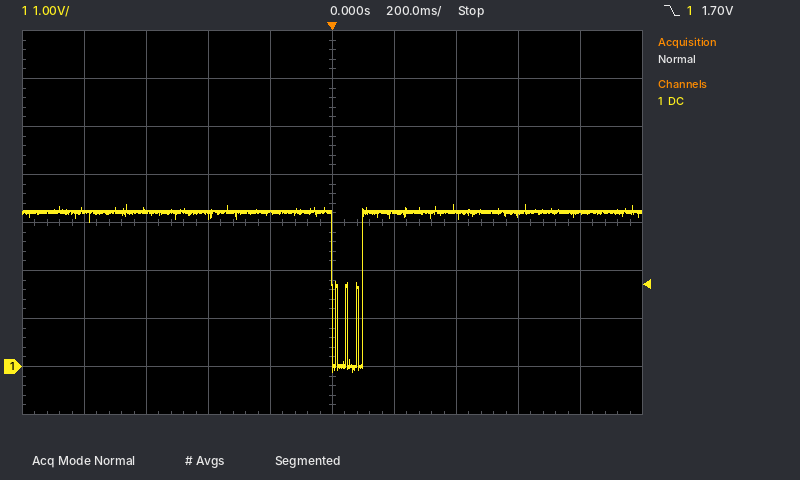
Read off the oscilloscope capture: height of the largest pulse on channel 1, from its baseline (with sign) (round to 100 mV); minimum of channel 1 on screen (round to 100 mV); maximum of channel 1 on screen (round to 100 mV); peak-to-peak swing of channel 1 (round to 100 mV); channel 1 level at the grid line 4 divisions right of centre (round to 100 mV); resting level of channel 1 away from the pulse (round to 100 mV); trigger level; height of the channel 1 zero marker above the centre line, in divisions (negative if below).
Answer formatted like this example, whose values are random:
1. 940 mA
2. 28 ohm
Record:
1. -3.3 V
2. -100 mV
3. 3.4 V
4. 3.5 V
5. 3.2 V
6. 3.2 V
7. 1.70 V
8. -3.0 div
